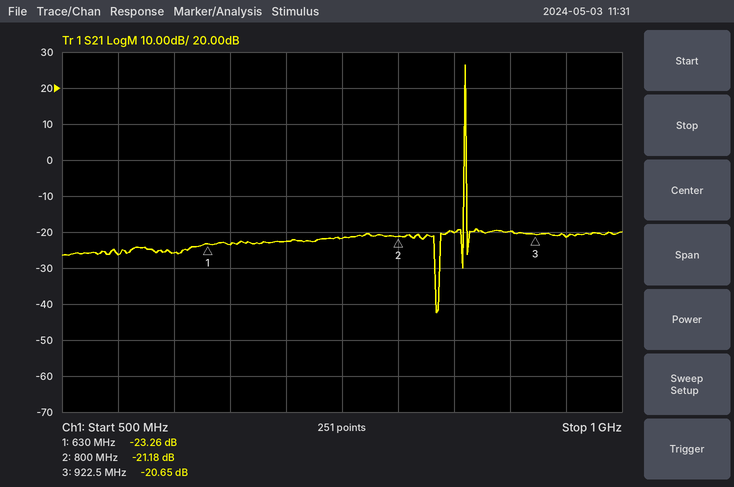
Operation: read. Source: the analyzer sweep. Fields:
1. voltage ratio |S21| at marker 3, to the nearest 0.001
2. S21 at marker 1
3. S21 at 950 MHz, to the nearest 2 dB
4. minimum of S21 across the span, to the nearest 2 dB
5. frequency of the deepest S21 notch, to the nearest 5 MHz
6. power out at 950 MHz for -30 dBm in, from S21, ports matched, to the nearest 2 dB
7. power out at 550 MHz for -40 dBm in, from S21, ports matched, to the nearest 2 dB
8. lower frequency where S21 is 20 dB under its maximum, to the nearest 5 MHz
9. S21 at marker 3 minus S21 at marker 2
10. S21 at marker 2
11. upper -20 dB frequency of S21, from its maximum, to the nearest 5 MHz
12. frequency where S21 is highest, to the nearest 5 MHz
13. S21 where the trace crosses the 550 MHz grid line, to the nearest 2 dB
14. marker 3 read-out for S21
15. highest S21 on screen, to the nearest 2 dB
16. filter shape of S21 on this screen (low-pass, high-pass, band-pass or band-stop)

0.093
-23.26 dB
-22 dB
-42 dB
835 MHz
-52 dBm
-66 dBm
860 MHz
0.53 dB
-21.18 dB
860 MHz
860 MHz
-26 dB
-20.65 dB
26 dB
band-pass
